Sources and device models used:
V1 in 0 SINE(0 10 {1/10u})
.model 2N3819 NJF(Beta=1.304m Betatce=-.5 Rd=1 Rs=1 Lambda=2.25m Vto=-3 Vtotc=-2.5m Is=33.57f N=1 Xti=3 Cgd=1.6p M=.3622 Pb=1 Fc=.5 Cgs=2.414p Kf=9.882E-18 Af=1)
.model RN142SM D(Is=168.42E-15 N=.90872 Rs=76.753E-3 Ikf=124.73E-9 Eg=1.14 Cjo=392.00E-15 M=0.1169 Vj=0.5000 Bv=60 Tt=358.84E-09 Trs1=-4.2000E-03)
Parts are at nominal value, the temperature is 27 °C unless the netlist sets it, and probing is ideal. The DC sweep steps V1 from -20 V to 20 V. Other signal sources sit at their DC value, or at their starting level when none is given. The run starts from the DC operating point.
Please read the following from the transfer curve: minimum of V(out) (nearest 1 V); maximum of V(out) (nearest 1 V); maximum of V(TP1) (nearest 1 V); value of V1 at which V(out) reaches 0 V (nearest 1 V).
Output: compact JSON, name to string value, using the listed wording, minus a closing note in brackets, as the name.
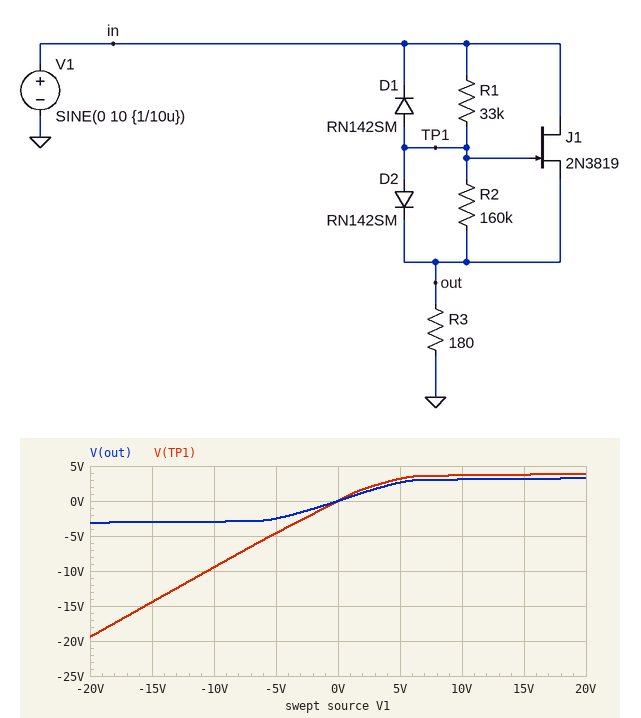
{"minimum of V(out)": "-3 V", "maximum of V(out)": "3 V", "maximum of V(TP1)": "4 V", "value of V1 at which V(out) reaches 0 V": "0 V"}
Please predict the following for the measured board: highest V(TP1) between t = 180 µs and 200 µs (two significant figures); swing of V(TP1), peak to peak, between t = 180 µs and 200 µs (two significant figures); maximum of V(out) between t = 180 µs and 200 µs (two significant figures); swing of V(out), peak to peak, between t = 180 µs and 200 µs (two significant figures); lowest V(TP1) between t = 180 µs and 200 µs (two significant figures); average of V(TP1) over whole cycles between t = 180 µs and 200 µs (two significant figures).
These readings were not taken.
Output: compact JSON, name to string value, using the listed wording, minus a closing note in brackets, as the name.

{"highest V(TP1) between t = 180 µs and 200 µs": "3.7 V", "swing of V(TP1), peak to peak, between t = 180 µs and 200 µs": "13 V", "maximum of V(out) between t = 180 µs and 200 µs": "3.1 V", "swing of V(out), peak to peak, between t = 180 µs and 200 µs": "6.0 V", "lowest V(TP1) between t = 180 µs and 200 µs": "-9.5 V", "average of V(TP1) over whole cycles between t = 180 µs and 200 µs": "-1.5 V"}
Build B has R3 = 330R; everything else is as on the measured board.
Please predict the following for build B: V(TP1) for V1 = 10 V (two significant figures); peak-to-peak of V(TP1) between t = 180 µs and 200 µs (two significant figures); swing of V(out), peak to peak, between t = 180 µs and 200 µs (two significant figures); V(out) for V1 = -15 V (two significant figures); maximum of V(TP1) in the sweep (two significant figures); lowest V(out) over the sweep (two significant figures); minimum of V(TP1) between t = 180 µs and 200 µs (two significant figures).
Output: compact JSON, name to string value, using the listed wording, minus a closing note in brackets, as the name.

{"V(TP1) for V1 = 10 V": "6.1 V", "peak-to-peak of V(TP1) between t = 180 µs and 200 µs": "16 V", "swing of V(out), peak to peak, between t = 180 µs and 200 µs": "11 V", "V(out) for V1 = -15 V": "-5.5 V", "maximum of V(TP1) in the sweep": "6.5 V", "lowest V(out) over the sweep": "-5.6 V", "minimum of V(TP1) between t = 180 µs and 200 µs": "-9.5 V"}
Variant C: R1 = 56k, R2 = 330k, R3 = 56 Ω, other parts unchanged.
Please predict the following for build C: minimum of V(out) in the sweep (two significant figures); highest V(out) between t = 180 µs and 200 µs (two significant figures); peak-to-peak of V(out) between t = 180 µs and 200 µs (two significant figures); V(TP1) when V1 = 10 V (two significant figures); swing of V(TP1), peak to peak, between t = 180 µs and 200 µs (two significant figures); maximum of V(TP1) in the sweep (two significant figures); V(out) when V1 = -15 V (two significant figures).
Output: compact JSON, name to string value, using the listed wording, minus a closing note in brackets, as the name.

{"minimum of V(out) in the sweep": "-950 mV", "highest V(out) between t = 180 µs and 200 µs": "960 mV", "peak-to-peak of V(out) between t = 180 µs and 200 µs": "1.9 V", "V(TP1) when V1 = 10 V": "1.5 V", "swing of V(TP1), peak to peak, between t = 180 µs and 200 µs": "11 V", "maximum of V(TP1) in the sweep": "1.6 V", "V(out) when V1 = -15 V": "-940 mV"}
